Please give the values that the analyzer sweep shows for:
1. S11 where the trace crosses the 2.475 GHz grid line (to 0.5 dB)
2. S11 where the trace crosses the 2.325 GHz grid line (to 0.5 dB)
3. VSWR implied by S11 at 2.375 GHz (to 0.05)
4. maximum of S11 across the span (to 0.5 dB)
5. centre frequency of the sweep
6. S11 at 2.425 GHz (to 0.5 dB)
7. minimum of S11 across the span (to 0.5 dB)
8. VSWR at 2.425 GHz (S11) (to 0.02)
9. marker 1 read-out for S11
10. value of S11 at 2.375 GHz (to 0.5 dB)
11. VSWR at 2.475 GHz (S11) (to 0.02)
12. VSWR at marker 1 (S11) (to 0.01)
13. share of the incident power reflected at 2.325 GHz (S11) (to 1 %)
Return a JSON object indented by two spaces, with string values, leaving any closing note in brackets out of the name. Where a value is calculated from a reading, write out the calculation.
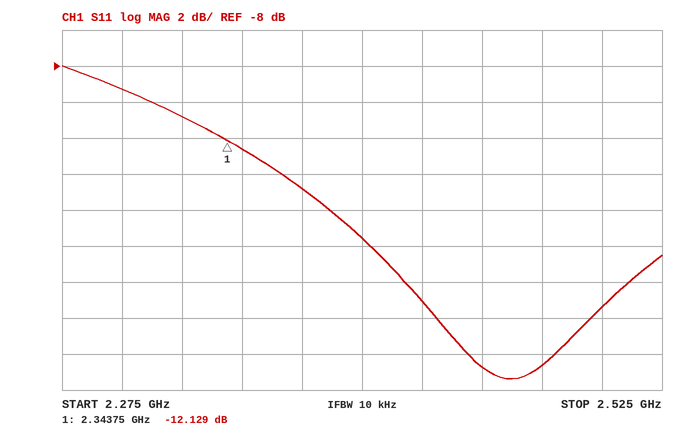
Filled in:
{
  "S11 where the trace crosses the 2.475 GHz grid line": "-24.5 dB",
  "S11 where the trace crosses the 2.325 GHz grid line": "-11.0 dB",
  "VSWR implied by S11 at 2.375 GHz": "|Γ| = 10^(-15/20) = 0.1778; VSWR = (1 + 0.1778)/(1 − 0.1778) ≈ 1.43, so 1.45 to the nearest 0.05",
  "maximum of S11 across the span": "-8.0 dB",
  "centre frequency of the sweep": "2.4 GHz",
  "S11 at 2.425 GHz": "-21.0 dB",
  "minimum of S11 across the span": "-25.5 dB",
  "VSWR at 2.425 GHz (S11)": "|Γ| = 10^(-21/20) = 0.0891; VSWR = (1 + 0.0891)/(1 − 0.0891) ≈ 1.20",
  "marker 1 read-out for S11": "-12.129 dB",
  "value of S11 at 2.375 GHz": "-15.0 dB",
  "VSWR at 2.475 GHz (S11)": "|Γ| = 10^(-24.5/20) = 0.0596; VSWR = (1 + 0.0596)/(1 − 0.0596) ≈ 1.13, so 1.12 to the nearest 0.02",
  "VSWR at marker 1 (S11)": "(1 + 0.2475)/(1 − 0.2475) ≈ 1.66",
  "share of the incident power reflected at 2.325 GHz (S11)": "10^(-11/10) ≈ 8 %"
}
